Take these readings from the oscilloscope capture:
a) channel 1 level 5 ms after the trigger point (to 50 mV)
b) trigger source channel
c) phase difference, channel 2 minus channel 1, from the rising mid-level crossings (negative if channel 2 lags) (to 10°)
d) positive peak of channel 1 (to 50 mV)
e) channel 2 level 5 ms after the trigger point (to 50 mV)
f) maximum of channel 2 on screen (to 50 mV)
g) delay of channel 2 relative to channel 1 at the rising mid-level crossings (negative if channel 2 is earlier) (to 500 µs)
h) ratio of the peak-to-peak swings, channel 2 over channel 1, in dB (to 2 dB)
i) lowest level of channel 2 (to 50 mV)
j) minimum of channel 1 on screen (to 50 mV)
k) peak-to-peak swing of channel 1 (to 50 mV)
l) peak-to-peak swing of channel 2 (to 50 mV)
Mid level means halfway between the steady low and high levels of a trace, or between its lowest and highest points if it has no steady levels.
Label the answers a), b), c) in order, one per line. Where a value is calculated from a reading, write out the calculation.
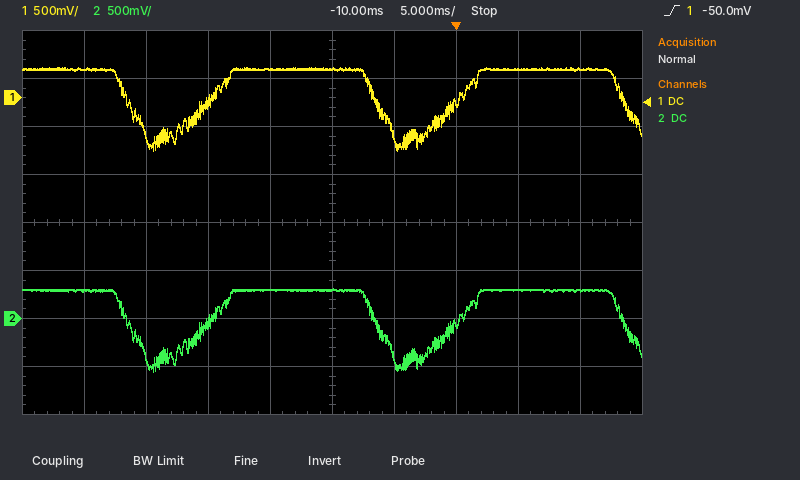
a) 300 mV
b) channel 1
c) 0°
d) 300 mV
e) 300 mV
f) 300 mV
g) 0.0 ms
h) 20 log10(850 mV / 850 mV) ≈ 0 dB
i) -550 mV
j) -550 mV
k) 300 mV − (-550 mV) = 850 mV
l) 300 mV − (-550 mV) = 850 mV
